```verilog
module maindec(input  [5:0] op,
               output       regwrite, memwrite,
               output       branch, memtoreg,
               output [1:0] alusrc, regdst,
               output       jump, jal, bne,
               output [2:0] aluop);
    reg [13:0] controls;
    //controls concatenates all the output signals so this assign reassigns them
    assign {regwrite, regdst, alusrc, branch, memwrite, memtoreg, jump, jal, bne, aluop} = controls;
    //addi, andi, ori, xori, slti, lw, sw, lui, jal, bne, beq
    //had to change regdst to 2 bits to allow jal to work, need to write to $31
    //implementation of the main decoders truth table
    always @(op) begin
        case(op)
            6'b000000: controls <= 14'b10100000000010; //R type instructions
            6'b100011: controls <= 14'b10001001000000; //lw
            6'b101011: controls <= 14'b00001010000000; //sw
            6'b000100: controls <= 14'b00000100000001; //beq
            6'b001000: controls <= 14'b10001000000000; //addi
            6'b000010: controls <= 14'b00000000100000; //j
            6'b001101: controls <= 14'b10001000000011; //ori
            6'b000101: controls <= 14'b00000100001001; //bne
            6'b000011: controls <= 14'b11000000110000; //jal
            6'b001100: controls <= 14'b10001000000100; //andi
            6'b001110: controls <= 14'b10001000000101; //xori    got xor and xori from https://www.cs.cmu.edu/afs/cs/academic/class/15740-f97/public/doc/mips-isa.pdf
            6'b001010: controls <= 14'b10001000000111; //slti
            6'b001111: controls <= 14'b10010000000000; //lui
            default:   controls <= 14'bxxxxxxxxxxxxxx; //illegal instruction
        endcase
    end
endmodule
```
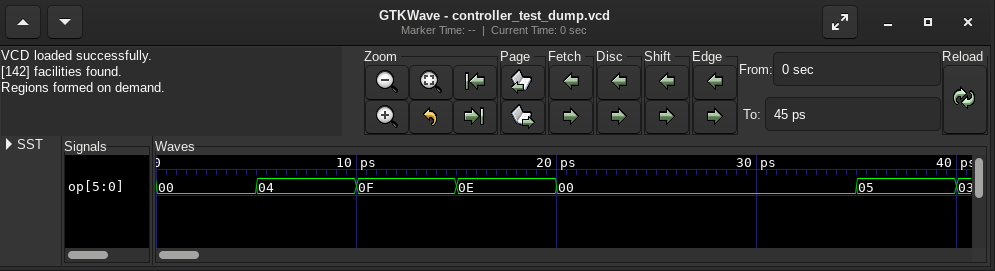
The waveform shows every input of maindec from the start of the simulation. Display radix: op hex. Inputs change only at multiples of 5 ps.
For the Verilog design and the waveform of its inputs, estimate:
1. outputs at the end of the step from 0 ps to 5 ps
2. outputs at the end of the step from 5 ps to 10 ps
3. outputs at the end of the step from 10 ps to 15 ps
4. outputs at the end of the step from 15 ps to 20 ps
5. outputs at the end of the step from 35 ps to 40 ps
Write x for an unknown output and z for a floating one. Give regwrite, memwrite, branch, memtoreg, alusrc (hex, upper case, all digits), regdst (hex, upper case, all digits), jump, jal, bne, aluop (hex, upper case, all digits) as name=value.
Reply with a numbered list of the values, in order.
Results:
1. regwrite=1, memwrite=0, branch=0, memtoreg=0, alusrc=0, regdst=1, jump=0, jal=0, bne=0, aluop=2
2. regwrite=0, memwrite=0, branch=1, memtoreg=0, alusrc=0, regdst=0, jump=0, jal=0, bne=0, aluop=1
3. regwrite=1, memwrite=0, branch=0, memtoreg=0, alusrc=2, regdst=0, jump=0, jal=0, bne=0, aluop=0
4. regwrite=1, memwrite=0, branch=0, memtoreg=0, alusrc=1, regdst=0, jump=0, jal=0, bne=0, aluop=5
5. regwrite=0, memwrite=0, branch=1, memtoreg=0, alusrc=0, regdst=0, jump=0, jal=0, bne=1, aluop=1
